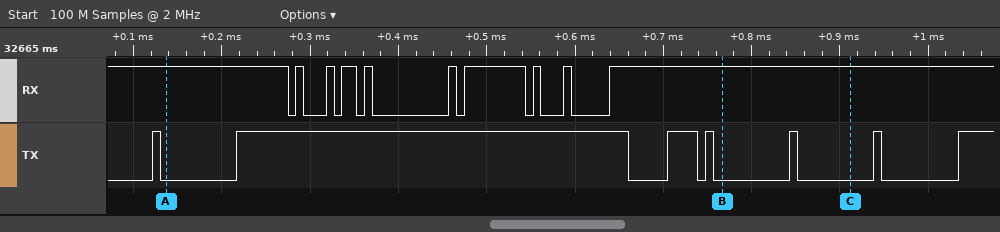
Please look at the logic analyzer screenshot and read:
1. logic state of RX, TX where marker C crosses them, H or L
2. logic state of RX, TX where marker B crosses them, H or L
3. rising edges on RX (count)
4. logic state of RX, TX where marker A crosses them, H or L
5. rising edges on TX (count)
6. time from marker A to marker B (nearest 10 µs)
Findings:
RX=H, TX=L
RX=H, TX=L
9
RX=H, TX=L
7
630 µs
